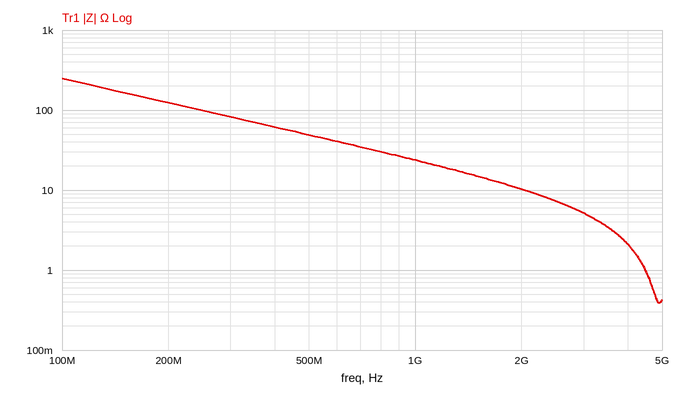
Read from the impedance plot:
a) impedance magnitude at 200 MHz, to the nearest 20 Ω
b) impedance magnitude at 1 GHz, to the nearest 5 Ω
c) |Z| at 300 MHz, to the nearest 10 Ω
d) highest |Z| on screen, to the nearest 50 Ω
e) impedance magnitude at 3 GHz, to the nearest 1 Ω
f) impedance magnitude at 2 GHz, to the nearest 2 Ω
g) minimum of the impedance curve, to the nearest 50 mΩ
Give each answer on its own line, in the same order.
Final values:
120 Ω
25 Ω
80 Ω
250 Ω
5 Ω
10 Ω
400 mΩ
